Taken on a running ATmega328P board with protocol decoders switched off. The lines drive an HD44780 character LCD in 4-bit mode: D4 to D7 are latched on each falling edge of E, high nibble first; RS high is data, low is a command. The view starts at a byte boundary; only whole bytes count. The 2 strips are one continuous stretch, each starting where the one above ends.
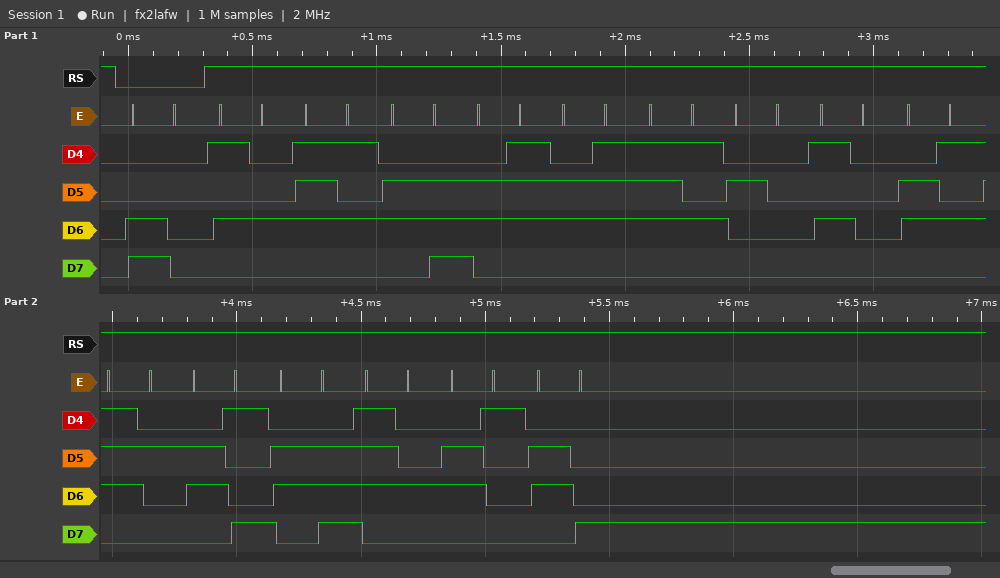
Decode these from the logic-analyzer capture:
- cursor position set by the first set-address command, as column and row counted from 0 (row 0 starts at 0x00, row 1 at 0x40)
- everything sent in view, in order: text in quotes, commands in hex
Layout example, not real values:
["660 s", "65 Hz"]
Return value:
["column 0, row 1", "0xC0 \"Tunggu Perintah\""]
